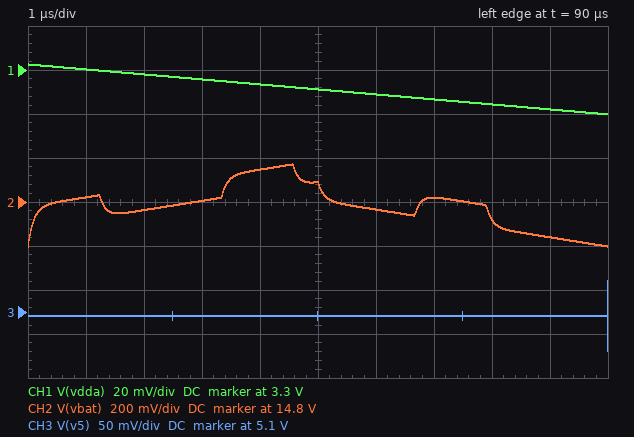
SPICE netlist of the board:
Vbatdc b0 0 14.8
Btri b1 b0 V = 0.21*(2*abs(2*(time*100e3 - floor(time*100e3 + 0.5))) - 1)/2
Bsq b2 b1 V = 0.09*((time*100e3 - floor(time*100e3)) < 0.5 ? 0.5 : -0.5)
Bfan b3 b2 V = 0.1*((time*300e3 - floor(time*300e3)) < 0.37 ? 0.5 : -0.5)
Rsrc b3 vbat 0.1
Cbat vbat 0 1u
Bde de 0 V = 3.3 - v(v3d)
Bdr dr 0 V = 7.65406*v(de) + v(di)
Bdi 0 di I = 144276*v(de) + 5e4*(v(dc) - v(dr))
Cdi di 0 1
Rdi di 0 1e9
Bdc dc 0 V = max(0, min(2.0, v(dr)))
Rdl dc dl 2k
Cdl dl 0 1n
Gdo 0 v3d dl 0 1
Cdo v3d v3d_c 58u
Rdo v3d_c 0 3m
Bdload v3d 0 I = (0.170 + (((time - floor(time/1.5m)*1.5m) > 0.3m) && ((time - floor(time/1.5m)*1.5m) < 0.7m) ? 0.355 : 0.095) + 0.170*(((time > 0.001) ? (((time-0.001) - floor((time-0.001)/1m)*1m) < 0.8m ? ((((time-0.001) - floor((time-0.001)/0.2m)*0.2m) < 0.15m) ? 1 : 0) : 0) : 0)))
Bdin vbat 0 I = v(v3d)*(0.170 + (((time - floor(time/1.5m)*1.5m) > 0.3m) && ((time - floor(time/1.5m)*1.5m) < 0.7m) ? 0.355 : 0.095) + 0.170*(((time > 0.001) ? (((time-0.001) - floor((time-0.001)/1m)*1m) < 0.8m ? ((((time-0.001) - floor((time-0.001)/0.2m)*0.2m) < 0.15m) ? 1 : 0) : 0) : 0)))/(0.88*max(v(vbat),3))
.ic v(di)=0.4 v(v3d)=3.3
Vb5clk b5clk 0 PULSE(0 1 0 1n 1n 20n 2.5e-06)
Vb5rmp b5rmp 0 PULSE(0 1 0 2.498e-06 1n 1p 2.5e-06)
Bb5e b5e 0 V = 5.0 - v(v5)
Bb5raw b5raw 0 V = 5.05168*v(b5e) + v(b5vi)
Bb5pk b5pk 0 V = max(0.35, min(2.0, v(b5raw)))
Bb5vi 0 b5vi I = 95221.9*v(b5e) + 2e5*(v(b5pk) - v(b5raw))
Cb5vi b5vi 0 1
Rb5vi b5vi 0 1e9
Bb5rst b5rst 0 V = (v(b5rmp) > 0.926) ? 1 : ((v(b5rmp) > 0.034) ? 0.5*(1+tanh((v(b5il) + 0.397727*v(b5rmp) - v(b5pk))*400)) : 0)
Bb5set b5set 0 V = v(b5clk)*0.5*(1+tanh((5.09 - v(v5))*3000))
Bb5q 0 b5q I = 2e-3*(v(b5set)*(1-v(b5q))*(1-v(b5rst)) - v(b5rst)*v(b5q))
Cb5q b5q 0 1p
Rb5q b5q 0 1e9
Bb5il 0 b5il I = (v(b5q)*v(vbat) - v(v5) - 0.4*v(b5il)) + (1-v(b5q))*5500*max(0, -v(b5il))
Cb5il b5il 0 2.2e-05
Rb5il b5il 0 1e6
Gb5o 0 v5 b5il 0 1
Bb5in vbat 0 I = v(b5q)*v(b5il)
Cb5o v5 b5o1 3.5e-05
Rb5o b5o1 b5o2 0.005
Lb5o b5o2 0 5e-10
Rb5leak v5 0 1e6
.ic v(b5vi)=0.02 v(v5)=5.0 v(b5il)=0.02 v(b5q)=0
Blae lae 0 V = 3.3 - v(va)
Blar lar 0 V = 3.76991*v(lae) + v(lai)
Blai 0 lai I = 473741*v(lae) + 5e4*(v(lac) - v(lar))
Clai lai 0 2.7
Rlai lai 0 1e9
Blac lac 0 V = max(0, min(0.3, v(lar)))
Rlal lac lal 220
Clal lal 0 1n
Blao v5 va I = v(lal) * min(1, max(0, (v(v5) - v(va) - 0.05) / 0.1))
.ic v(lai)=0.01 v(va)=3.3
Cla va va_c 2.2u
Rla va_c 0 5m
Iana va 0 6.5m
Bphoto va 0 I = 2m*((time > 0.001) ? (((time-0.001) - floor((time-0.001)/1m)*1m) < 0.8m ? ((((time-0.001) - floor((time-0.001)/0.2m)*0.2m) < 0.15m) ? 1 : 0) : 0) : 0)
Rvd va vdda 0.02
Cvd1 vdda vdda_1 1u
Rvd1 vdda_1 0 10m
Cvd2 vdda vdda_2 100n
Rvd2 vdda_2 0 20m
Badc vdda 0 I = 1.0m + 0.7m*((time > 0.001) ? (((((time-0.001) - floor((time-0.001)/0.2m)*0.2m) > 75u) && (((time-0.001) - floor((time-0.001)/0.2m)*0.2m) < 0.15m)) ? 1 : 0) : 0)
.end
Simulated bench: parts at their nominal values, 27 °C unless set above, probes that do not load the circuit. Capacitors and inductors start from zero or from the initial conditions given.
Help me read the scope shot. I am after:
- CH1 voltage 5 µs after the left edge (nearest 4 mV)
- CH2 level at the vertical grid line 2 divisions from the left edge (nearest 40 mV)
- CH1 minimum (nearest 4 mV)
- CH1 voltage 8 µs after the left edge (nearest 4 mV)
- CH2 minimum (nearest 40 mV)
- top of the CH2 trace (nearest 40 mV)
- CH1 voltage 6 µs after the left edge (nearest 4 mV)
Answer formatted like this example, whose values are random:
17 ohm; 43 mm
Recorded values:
3.292 V; 14.76 V; 3.280 V; 3.284 V; 14.60 V; 14.96 V; 3.288 V
